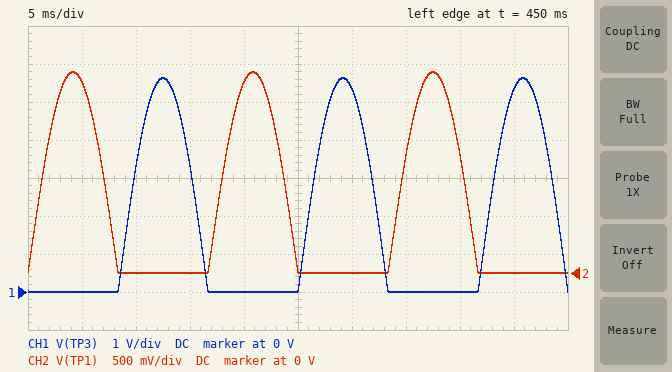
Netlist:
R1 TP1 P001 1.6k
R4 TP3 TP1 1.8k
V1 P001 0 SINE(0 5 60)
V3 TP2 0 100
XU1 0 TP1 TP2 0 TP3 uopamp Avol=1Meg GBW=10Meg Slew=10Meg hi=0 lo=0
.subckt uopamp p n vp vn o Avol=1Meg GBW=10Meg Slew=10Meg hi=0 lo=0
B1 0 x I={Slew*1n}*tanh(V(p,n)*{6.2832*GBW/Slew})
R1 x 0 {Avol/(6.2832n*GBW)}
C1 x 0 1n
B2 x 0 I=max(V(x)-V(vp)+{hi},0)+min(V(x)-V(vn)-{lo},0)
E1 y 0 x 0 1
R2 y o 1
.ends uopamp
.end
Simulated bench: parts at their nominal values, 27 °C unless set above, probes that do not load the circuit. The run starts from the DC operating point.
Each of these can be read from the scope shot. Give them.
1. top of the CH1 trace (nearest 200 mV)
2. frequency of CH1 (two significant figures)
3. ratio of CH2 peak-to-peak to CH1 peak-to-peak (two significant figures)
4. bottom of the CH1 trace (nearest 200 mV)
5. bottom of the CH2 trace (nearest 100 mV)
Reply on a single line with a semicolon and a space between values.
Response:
5.6 V; 60 Hz; 0.47; 0 V; 0 V
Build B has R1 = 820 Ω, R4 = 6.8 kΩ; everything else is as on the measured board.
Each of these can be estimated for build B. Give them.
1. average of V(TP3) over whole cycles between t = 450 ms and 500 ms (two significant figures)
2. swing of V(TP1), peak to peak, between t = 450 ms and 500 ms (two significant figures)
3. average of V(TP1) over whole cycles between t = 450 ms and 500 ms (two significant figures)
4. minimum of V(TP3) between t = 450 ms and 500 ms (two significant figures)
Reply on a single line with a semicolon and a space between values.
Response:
13 V; 4.5 V; 1.4 V; -9.9 mV
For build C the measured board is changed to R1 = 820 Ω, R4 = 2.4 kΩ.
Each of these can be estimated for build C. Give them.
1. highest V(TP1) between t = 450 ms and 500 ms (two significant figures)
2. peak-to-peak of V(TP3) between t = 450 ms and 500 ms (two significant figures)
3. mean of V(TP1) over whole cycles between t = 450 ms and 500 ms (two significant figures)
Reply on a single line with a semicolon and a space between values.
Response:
3.7 V; 15 V; 1.2 V
